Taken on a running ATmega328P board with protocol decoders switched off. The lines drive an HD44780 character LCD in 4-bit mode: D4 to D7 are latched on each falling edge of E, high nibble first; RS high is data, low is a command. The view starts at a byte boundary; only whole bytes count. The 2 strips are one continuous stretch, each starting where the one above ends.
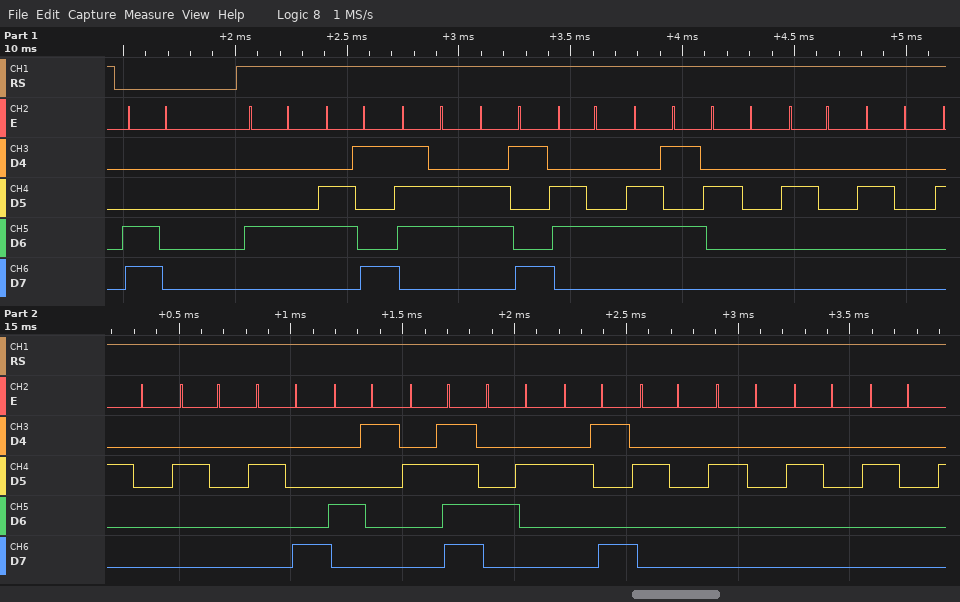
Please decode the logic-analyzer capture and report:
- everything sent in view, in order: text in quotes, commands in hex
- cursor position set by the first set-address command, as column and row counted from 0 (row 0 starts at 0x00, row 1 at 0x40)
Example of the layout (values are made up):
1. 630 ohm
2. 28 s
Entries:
1. 0xC0 "Divide     (A/B)    "
2. column 0, row 1
